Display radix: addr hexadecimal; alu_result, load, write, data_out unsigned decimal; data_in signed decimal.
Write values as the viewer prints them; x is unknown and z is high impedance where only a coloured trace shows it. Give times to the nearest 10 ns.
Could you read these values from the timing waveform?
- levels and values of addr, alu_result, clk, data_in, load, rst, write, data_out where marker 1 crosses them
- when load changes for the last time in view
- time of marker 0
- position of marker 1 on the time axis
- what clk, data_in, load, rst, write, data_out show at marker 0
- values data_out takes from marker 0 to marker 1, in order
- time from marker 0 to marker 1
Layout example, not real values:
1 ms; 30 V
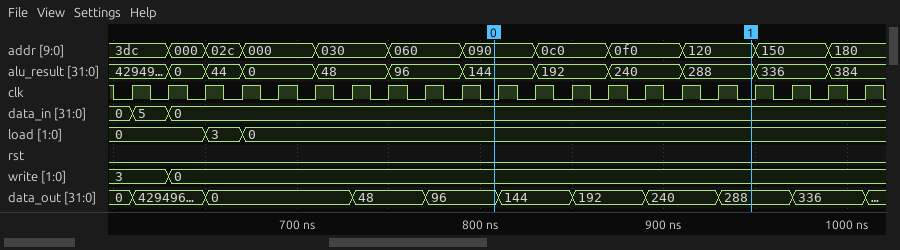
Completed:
addr=120, alu_result=288, clk=0, data_in=0, load=0, rst=0, write=0, data_out=288; 670 ns; 810 ns; 950 ns; clk=0, data_in=0, load=0, rst=0, write=0, data_out=96; 96, 144, 192, 240, 288; 140 ns
